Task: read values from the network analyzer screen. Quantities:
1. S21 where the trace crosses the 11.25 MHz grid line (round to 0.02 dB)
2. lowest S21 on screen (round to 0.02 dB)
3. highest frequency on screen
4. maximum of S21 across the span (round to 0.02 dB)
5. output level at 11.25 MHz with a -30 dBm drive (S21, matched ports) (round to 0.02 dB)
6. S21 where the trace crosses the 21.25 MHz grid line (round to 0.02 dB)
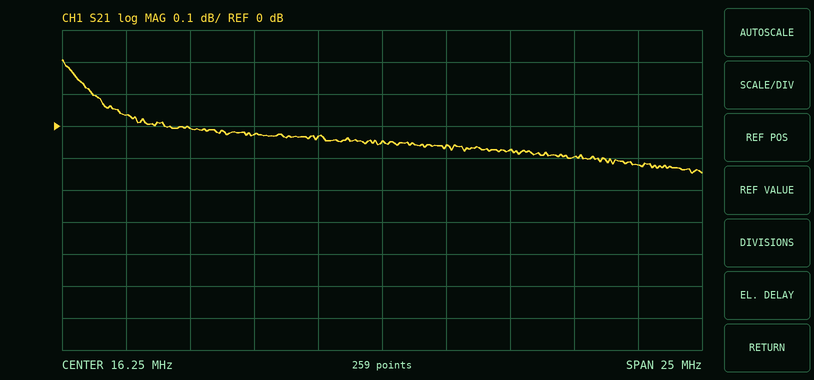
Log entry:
-0.02 dB
-0.14 dB
28.75 MHz
0.20 dB
-30.02 dBm
-0.08 dB
